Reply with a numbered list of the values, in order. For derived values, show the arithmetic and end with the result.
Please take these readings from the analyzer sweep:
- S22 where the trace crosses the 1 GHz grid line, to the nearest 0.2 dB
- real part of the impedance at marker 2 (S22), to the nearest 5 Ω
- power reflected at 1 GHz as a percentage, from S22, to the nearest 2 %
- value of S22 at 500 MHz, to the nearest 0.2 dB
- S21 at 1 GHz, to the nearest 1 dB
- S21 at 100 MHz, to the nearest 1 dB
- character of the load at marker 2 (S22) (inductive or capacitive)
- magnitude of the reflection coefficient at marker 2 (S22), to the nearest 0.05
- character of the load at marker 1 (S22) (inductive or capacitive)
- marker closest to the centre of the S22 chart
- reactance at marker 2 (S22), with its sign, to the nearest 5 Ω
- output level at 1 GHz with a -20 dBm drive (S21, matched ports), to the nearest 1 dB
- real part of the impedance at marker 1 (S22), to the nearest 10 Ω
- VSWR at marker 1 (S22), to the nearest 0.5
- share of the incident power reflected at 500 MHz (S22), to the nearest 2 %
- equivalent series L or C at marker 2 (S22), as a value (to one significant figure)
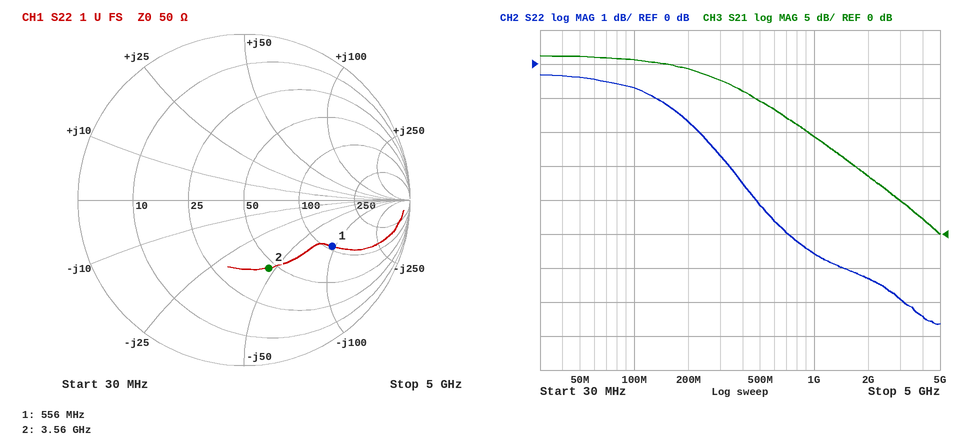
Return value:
1. -5.6 dB
2. 45 Ω
3. 10^(-5.6/10) ≈ 28 %
4. -4.2 dB
5. 14 dB
6. 26 dB
7. capacitive
8. 0.45
9. capacitive
10. marker 2
11. -45 Ω
12. -20 dBm + (14 dB) = -6 dBm
13. 110 Ω
14. 4.0
15. 10^(-4.2/10) ≈ 38 %
16. C = 1/(2π × 3.56 GHz × 45 Ω) ≈ 1.0 pF
